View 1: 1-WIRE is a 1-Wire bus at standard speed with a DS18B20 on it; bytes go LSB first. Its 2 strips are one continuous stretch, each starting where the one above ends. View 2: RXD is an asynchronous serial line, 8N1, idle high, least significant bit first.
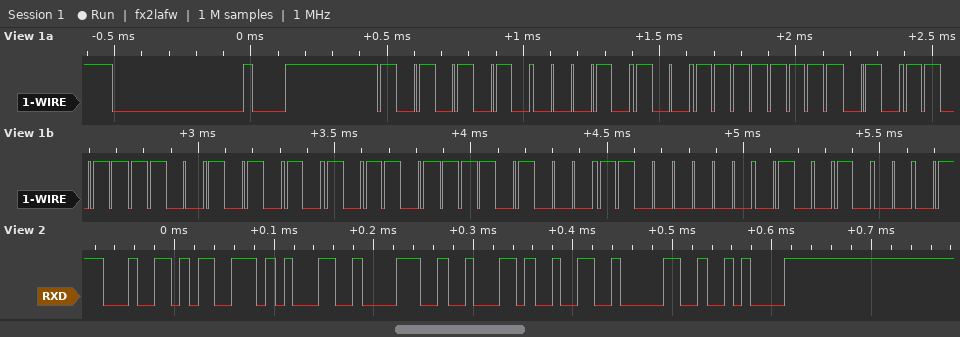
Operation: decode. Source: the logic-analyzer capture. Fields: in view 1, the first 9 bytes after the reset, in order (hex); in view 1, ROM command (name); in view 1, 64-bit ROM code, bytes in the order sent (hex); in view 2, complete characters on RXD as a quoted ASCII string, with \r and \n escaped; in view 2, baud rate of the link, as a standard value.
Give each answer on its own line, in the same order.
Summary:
55 28 FF DA 53 B5 17 03 12
Match ROM
28 FF DA 53 B5 17 03 12
"ds18b20\n"
115200 baud
